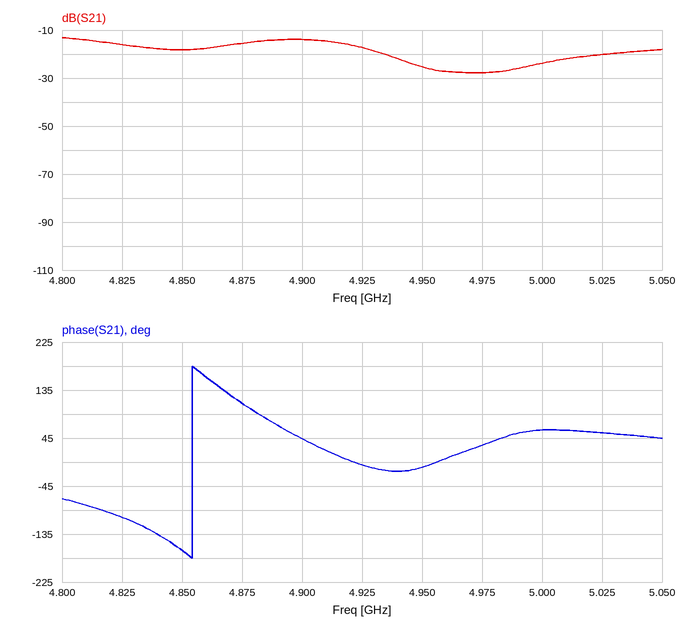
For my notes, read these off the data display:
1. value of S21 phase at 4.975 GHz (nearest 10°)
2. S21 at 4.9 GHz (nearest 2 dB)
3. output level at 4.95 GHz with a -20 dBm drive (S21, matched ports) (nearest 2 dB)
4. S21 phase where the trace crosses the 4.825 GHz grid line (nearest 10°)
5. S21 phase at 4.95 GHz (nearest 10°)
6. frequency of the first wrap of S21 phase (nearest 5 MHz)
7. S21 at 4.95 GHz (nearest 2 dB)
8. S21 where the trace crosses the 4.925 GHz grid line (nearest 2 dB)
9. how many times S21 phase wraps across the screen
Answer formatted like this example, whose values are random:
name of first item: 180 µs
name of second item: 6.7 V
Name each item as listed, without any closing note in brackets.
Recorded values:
value of S21 phase at 4.975 GHz: 30°
S21 at 4.9 GHz: -14 dB
output level at 4.95 GHz with a -20 dBm drive (S21, matched ports): -46 dBm
S21 phase where the trace crosses the 4.825 GHz grid line: -100°
S21 phase at 4.95 GHz: -10°
frequency of the first wrap of S21 phase: 4.855 GHz
S21 at 4.95 GHz: -26 dB
S21 where the trace crosses the 4.925 GHz grid line: -18 dB
how many times S21 phase wraps across the screen: 1
